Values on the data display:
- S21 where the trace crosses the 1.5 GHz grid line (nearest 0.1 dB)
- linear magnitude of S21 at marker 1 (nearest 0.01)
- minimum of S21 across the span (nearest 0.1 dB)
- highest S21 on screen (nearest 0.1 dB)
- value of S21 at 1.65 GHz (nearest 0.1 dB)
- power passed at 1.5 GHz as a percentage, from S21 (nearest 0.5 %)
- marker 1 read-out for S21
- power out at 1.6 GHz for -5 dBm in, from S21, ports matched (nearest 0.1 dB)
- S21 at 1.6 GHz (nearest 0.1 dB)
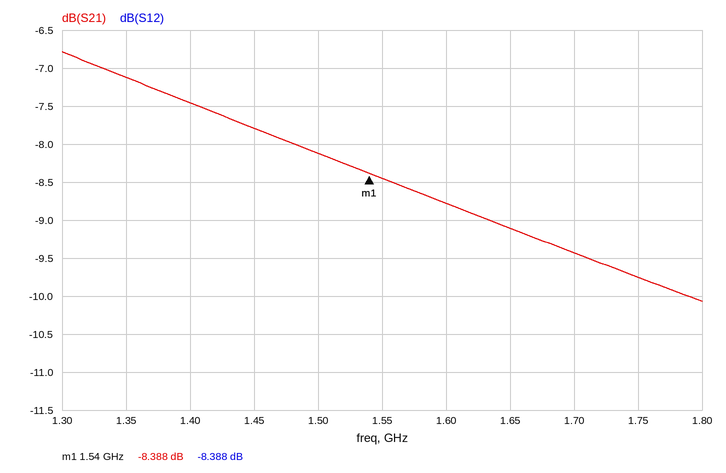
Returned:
-8.1 dB
0.38
-10.1 dB
-6.8 dB
-9.1 dB
15.5 %
-8.388 dB
-13.8 dBm
-8.8 dB
